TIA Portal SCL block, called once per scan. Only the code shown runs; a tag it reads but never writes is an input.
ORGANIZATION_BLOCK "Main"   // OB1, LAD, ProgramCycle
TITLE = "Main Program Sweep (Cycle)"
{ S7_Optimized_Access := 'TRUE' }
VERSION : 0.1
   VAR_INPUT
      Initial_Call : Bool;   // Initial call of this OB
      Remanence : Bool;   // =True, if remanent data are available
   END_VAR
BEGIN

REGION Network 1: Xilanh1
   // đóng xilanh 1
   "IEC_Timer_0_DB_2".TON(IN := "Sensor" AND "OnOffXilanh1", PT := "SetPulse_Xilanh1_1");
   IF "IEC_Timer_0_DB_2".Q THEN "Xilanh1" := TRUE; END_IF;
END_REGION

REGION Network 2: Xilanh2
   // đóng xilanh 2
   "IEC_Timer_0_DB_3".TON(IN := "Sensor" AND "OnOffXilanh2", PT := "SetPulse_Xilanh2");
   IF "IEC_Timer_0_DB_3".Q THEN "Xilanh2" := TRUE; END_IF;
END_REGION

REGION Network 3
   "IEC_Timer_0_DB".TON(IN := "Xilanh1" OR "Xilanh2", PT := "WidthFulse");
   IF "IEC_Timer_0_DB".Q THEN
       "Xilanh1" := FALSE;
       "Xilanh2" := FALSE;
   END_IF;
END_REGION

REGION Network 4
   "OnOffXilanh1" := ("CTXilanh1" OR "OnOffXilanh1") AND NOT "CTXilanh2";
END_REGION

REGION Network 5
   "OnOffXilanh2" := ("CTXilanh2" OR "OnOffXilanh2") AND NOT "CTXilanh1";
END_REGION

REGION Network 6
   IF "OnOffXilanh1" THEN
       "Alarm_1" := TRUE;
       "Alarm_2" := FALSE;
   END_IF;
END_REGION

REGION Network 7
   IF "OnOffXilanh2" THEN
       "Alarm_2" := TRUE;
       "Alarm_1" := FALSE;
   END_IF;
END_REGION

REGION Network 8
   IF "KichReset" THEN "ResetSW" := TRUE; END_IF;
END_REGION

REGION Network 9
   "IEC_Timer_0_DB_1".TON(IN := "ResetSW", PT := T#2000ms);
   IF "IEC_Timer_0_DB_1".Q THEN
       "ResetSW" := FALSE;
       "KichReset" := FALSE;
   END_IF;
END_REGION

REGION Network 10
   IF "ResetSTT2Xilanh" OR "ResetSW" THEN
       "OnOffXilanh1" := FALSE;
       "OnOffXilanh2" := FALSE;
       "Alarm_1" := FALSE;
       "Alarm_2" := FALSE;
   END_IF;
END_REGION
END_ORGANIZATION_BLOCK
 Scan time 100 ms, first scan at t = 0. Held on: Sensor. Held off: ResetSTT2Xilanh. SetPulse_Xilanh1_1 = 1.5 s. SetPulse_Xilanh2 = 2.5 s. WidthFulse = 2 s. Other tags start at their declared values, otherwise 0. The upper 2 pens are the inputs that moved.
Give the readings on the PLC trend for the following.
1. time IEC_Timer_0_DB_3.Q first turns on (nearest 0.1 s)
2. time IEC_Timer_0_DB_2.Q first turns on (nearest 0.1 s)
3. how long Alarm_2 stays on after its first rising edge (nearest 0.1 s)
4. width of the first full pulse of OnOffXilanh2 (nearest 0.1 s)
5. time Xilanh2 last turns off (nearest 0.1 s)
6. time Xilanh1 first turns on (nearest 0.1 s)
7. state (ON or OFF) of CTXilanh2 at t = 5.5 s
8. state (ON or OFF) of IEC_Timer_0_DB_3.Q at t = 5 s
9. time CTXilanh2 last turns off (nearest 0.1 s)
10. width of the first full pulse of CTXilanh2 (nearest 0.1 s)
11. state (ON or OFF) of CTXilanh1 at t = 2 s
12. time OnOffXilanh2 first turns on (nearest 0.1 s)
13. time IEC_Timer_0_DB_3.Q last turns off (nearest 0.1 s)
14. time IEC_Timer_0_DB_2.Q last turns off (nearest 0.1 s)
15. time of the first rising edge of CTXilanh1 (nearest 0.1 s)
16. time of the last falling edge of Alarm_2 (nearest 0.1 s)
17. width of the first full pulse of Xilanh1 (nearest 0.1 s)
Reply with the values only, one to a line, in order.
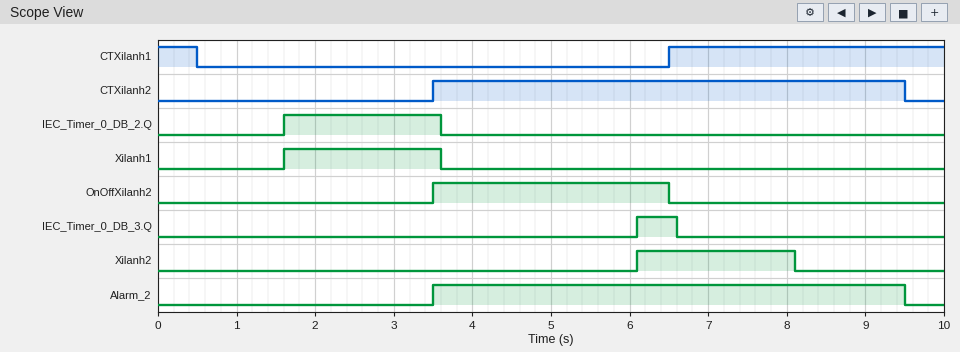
6.1 s
1.6 s
6.0 s
3.0 s
8.1 s
1.6 s
ON
OFF
9.5 s
6.0 s
OFF
3.5 s
6.6 s
3.6 s
6.5 s
9.5 s
2.0 s
